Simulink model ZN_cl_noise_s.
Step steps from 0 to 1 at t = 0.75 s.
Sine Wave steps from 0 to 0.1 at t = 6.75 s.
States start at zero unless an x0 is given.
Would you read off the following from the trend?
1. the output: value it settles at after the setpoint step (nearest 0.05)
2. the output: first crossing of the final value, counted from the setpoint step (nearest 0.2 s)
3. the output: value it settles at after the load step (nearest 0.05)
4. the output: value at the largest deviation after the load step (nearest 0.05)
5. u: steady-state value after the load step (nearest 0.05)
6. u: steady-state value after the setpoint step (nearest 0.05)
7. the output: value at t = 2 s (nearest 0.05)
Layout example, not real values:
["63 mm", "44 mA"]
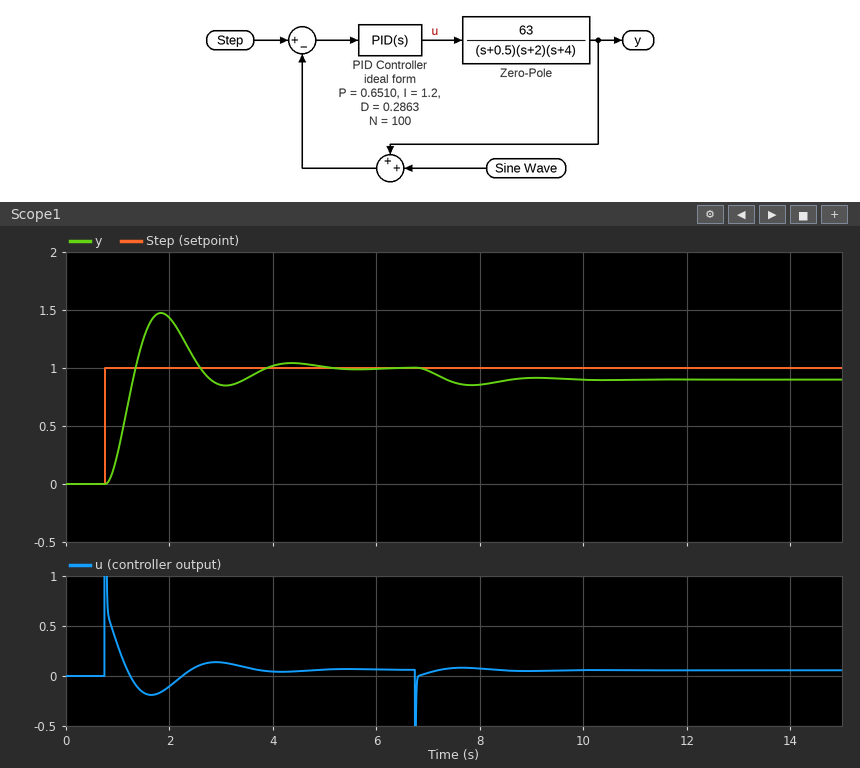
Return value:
["1.00", "0.6 s", "0.90", "0.85", "0.05", "0.05", "1.45"]
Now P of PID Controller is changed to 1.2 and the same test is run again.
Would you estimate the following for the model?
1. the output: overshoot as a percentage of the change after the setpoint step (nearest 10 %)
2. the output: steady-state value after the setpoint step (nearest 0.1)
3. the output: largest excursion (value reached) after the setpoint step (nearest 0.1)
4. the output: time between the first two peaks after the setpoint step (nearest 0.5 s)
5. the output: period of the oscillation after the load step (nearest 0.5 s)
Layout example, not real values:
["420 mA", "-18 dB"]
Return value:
["50 %", "1.0", "1.5", "1.5 s", "1.5 s"]
